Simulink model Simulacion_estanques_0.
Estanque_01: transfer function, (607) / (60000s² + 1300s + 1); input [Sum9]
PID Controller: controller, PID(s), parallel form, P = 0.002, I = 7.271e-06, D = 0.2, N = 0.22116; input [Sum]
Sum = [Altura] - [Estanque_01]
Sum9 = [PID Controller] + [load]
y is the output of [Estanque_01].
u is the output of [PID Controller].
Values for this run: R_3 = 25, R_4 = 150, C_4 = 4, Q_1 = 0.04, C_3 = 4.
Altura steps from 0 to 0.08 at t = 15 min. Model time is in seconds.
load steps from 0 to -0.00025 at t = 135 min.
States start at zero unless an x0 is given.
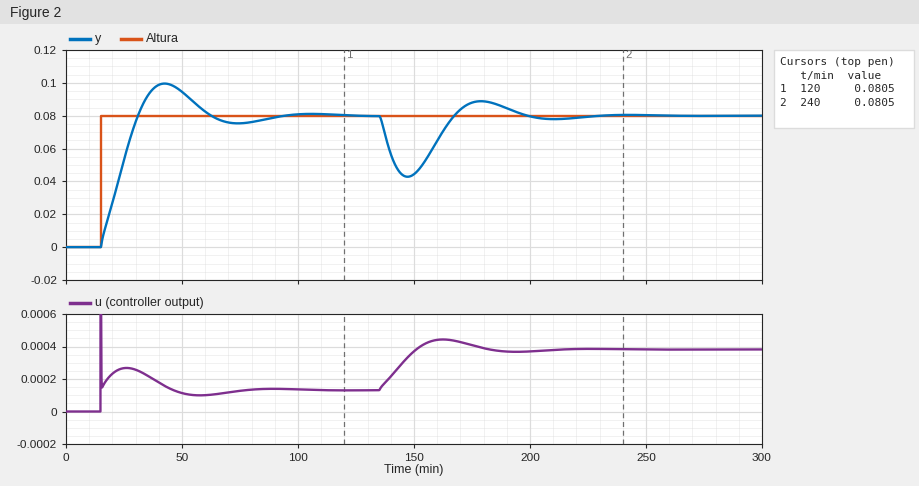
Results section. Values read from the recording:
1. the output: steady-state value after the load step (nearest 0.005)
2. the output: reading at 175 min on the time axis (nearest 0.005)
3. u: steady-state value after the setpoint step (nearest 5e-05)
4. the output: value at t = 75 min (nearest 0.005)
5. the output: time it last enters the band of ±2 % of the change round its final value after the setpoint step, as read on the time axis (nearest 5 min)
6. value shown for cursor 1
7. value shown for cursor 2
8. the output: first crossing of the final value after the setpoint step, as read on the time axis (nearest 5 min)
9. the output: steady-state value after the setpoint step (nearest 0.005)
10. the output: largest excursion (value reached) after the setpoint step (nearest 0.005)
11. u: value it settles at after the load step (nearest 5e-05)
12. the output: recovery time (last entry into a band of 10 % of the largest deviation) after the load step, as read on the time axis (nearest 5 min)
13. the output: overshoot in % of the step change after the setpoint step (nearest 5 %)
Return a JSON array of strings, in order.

["0.080", "0.090", "0.00015", "0.075", "90 min", "0.0805", "0.0805", "30 min", "0.080", "0.100", "0.00040", "190 min", "25 %"]
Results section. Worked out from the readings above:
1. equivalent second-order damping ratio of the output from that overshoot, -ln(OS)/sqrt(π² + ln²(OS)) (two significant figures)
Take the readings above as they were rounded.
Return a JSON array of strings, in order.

["0.40"]
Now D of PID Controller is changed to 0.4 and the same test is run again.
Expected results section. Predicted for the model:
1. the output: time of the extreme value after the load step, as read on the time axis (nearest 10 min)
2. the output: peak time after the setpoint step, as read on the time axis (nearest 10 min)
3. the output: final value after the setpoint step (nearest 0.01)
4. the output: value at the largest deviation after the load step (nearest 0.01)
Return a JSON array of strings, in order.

["150 min", "40 min", "0.08", "0.04"]
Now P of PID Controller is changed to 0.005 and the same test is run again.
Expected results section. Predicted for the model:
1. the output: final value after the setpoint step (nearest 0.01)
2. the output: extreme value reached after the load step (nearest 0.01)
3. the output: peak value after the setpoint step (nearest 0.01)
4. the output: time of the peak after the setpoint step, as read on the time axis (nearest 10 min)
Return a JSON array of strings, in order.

["0.08", "0.05", "0.09", "40 min"]
